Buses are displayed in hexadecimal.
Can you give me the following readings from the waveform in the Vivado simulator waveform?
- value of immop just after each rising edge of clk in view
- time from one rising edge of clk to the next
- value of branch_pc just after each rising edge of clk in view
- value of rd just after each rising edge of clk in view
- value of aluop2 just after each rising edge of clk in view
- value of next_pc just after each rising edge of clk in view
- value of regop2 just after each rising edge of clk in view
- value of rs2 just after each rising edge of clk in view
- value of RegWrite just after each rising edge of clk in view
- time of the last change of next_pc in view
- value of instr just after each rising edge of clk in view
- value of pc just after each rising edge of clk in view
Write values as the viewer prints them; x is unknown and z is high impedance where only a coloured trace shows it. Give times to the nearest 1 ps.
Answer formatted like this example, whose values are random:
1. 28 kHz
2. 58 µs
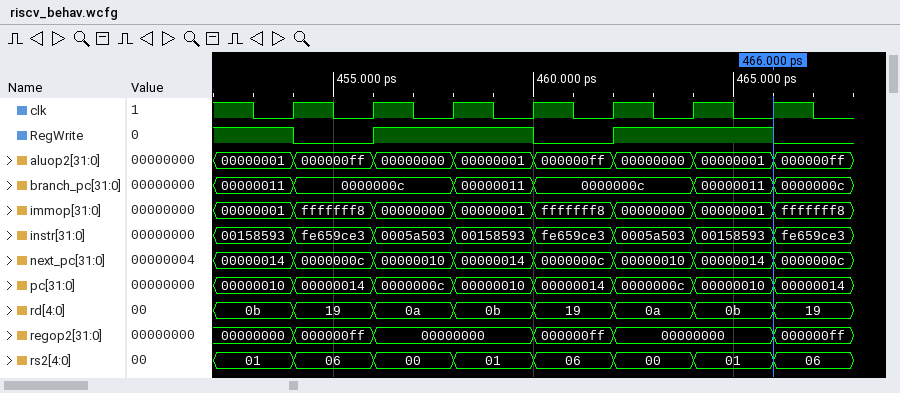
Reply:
1. fffffff8, 00000000, 00000001, fffffff8, 00000000, 00000001, fffffff8
2. 2 ps
3. 0000000c, 0000000c, 00000011, 0000000c, 0000000c, 00000011, 0000000c
4. 19, 0a, 0b, 19, 0a, 0b, 19
5. 000000ff, 00000000, 00000001, 000000ff, 00000000, 00000001, 000000ff
6. 0000000c, 00000010, 00000014, 0000000c, 00000010, 00000014, 0000000c
7. 000000ff, 00000000, 00000000, 000000ff, 00000000, 00000000, 000000ff
8. 06, 00, 01, 06, 00, 01, 06
9. 0 1 1 0 1 1 0
10. 466 ps
11. fe659ce3, 0005a503, 00158593, fe659ce3, 0005a503, 00158593, fe659ce3
12. 00000014, 0000000c, 00000010, 00000014, 0000000c, 00000010, 00000014
